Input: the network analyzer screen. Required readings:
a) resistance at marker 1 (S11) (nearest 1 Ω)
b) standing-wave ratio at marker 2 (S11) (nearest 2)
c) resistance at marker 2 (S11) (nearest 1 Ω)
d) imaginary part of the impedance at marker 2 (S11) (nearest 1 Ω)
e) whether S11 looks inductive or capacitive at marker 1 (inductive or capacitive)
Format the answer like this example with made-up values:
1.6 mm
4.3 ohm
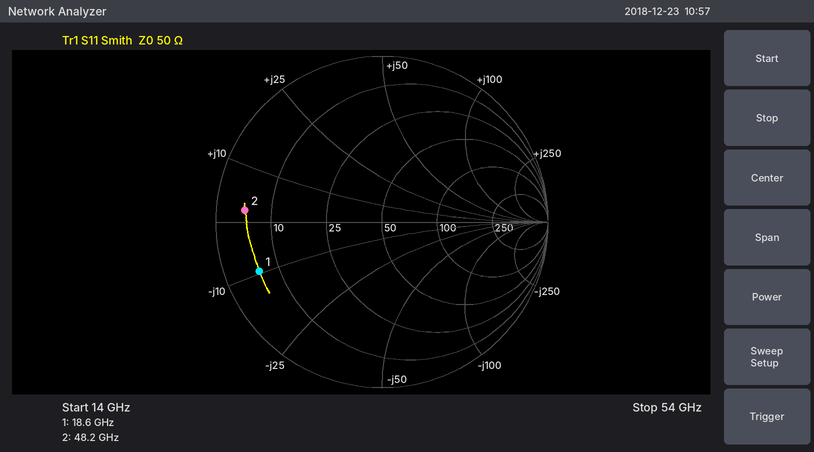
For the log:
6 Ω
10
5 Ω
+2 Ω
capacitive
